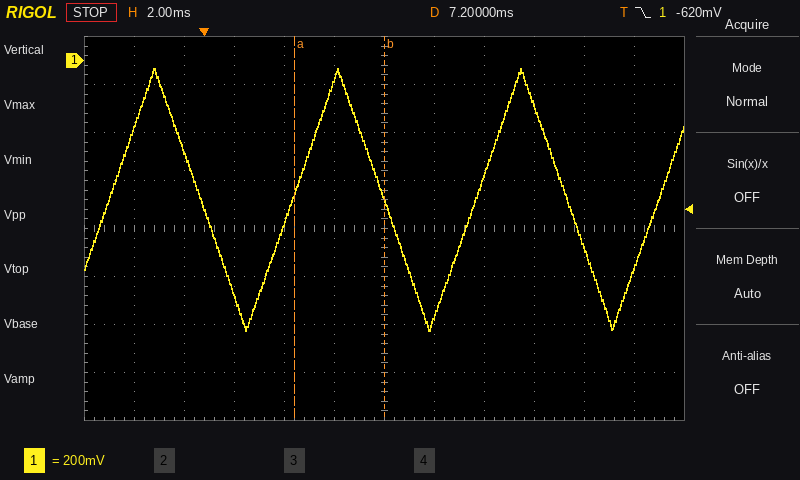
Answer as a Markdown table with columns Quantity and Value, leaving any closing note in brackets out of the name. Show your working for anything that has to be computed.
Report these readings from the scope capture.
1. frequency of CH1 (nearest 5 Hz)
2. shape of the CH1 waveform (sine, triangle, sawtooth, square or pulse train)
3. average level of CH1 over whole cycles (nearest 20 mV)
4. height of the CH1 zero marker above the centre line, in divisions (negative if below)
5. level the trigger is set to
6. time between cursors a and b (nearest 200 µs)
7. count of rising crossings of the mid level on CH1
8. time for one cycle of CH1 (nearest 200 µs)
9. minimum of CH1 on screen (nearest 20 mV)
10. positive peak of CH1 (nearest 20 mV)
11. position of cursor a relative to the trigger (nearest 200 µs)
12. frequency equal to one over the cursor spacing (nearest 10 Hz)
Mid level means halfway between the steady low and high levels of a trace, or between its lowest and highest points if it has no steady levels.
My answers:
| Quantity | Value |
|---|---|
| frequency of CH1 | 1 / 7.4 ms ≈ 135 Hz |
| shape of the CH1 waveform | triangle |
| average level of CH1 over whole cycles | (-40 mV + (-1.12 V)) / 2 ≈ -580 mV |
| height of the CH1 zero marker above the centre line, in divisions | +3.5 div |
| level the trigger is set to | -620 mV |
| time between cursors a and b | 3.6 ms |
| count of rising crossings of the mid level on CH1 | 4 |
| time for one cycle of CH1 | 7.4 ms |
| minimum of CH1 on screen | -1.12 V |
| positive peak of CH1 | -40 mV |
| position of cursor a relative to the trigger | +3.6 ms |
| frequency equal to one over the cursor spacing | 1 / 3.6 ms ≈ 280 Hz |
